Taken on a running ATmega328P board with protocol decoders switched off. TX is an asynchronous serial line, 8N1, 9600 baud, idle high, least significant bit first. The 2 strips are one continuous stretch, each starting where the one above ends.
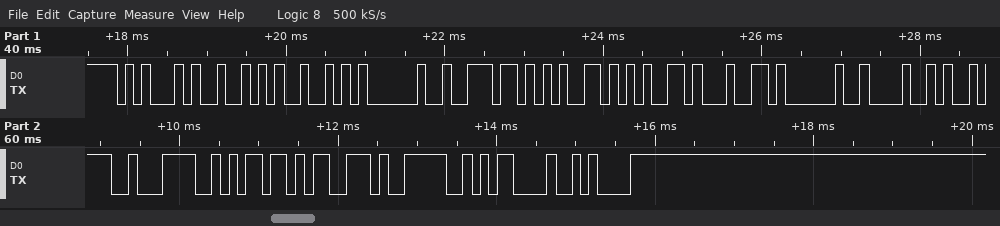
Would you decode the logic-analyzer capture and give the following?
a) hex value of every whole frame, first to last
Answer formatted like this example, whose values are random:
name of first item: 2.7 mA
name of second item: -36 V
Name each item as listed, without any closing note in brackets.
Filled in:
hex value of every whole frame, first to last: 0x45 0x52 0x52 0x20 0x6E 0x65 0x65 0x64 0x20 0x48 0x3A 0x3C 0x6D 0x73 0x3E 0x0D 0x0A
